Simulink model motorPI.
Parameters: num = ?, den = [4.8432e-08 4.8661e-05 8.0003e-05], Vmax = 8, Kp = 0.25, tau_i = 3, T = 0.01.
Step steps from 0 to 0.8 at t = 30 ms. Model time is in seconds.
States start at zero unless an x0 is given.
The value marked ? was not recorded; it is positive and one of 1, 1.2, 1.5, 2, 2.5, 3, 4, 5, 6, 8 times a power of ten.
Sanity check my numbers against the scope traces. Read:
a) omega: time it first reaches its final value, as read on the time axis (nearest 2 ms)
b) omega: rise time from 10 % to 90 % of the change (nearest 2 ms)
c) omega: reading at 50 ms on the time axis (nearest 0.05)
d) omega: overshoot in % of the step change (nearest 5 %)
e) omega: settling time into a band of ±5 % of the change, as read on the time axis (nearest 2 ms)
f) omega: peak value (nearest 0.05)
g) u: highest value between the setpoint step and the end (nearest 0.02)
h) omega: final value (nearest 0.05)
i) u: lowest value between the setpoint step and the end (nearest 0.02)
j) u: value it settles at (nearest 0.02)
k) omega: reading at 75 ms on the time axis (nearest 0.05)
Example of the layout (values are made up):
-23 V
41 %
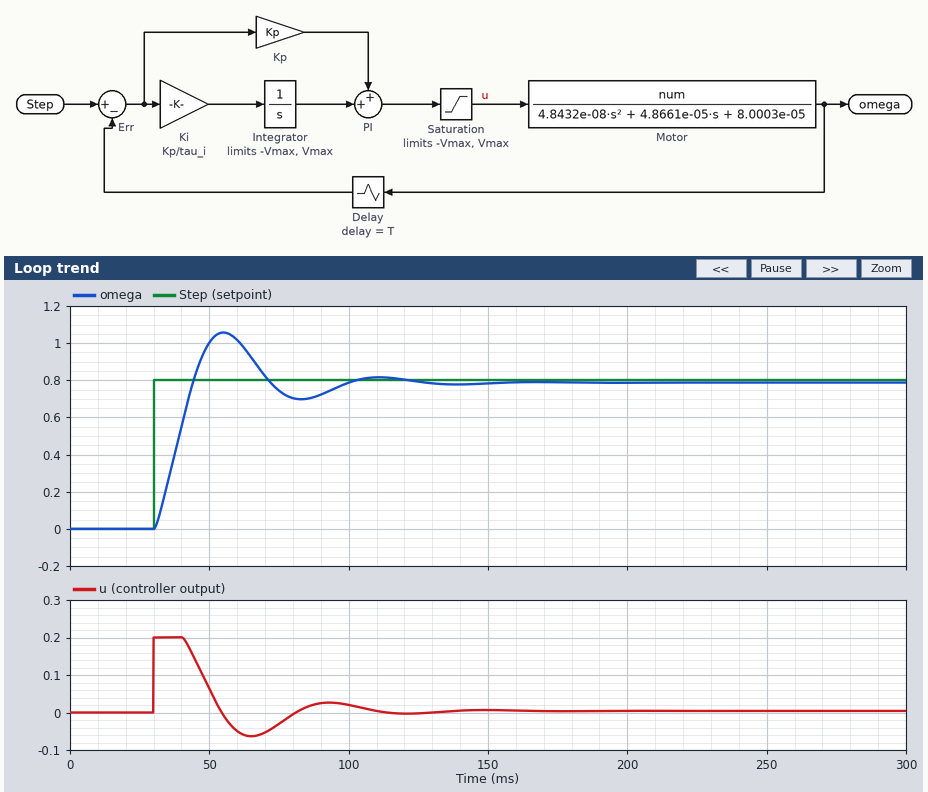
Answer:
44 ms
10 ms
1.00
35 %
94 ms
1.05
0.20
0.80
-0.06
0.00
0.75
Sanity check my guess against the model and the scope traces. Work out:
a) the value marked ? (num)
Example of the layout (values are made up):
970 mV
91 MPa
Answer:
0.015
